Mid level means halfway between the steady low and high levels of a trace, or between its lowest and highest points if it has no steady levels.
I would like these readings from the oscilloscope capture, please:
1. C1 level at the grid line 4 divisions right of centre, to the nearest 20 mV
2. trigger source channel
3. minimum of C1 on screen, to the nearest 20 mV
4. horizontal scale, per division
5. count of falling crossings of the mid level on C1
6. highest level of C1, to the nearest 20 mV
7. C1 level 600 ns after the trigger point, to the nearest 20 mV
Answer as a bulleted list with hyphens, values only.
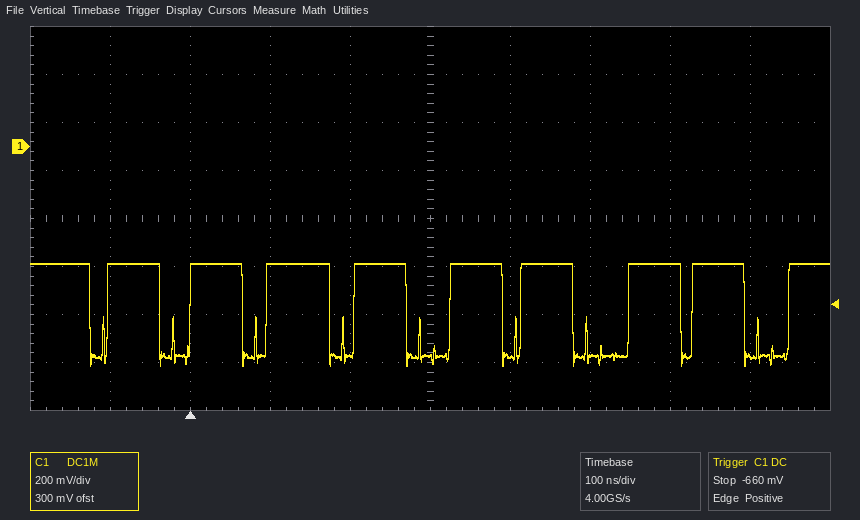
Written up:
- -880 mV
- C1
- -920 mV
- 100 ns
- 9
- -480 mV
- -480 mV
